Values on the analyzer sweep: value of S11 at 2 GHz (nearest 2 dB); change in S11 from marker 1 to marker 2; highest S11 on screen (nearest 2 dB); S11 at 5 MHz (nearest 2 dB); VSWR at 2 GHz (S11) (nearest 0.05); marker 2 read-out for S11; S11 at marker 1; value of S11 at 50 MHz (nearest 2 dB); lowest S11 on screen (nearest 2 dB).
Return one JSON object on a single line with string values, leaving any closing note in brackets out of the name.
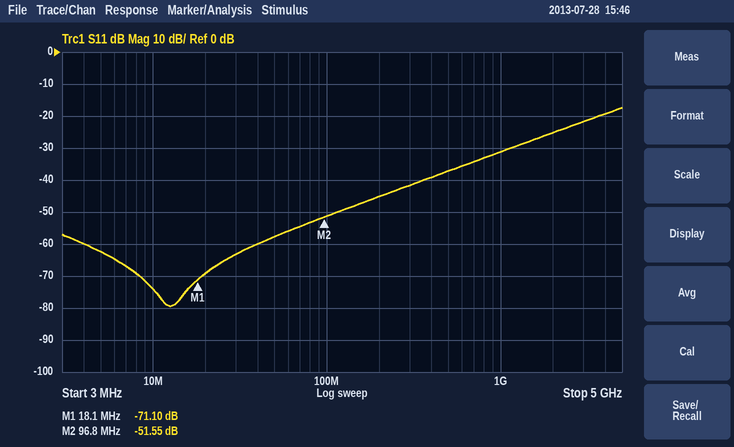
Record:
{"value of S11 at 2 GHz": "-26 dB", "change in S11 from marker 1 to marker 2": "19.55 dB", "highest S11 on screen": "-18 dB", "S11 at 5 MHz": "-62 dB", "VSWR at 2 GHz (S11)": "1.10", "marker 2 read-out for S11": "-51.55 dB", "S11 at marker 1": "-71.10 dB", "value of S11 at 50 MHz": "-58 dB", "lowest S11 on screen": "-80 dB"}
